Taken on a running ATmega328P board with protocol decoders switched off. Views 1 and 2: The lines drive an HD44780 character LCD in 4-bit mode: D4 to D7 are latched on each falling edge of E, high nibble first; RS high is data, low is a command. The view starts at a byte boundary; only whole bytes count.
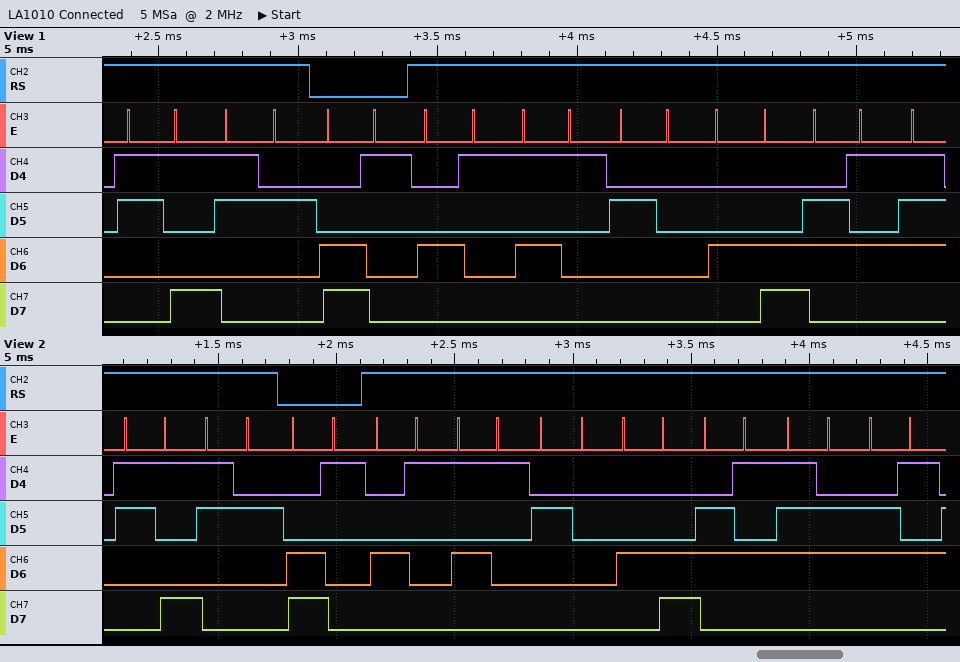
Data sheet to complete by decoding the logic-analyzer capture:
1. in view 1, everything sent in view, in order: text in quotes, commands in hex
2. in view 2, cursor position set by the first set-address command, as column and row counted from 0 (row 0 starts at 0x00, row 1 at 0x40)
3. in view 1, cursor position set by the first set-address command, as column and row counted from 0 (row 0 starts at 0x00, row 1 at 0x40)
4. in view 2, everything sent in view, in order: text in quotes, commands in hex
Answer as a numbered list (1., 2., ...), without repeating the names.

1. "92" 0xC1 "AQ Le"
2. column 1, row 1
3. column 1, row 1
4. "92" 0xC1 "AQ Leve"
